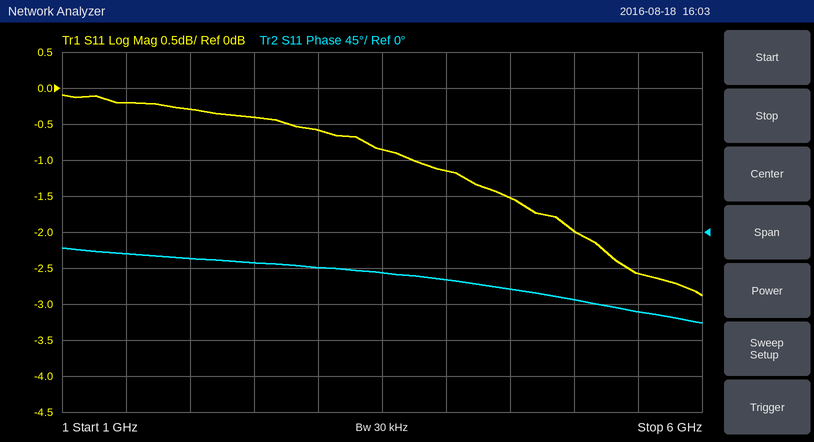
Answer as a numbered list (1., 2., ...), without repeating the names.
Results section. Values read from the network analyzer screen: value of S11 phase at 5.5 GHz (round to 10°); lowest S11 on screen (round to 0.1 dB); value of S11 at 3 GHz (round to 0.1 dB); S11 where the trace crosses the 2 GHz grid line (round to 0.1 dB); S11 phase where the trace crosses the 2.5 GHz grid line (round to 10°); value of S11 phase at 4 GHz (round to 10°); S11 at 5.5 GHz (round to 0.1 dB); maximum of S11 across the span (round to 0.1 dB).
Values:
1. -100°
2. -2.9 dB
3. -0.6 dB
4. -0.3 dB
5. -40°
6. -60°
7. -2.6 dB
8. -0.1 dB
